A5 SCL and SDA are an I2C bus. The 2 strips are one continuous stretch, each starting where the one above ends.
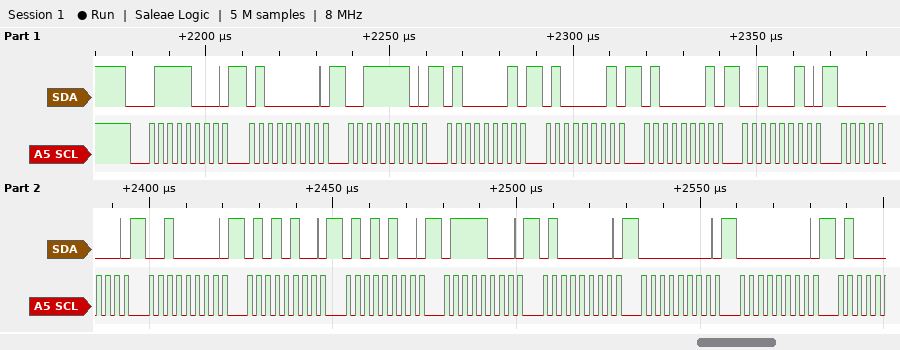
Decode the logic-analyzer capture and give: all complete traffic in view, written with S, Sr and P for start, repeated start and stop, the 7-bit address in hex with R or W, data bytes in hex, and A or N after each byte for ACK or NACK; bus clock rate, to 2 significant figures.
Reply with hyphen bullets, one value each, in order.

- S 3CW A 40 A 3E A 41 A 41 A 41 A 22 A 00 A 20 A 54 A 54 A 78 A 40 A 00 A 00 A
- 400 kHz
